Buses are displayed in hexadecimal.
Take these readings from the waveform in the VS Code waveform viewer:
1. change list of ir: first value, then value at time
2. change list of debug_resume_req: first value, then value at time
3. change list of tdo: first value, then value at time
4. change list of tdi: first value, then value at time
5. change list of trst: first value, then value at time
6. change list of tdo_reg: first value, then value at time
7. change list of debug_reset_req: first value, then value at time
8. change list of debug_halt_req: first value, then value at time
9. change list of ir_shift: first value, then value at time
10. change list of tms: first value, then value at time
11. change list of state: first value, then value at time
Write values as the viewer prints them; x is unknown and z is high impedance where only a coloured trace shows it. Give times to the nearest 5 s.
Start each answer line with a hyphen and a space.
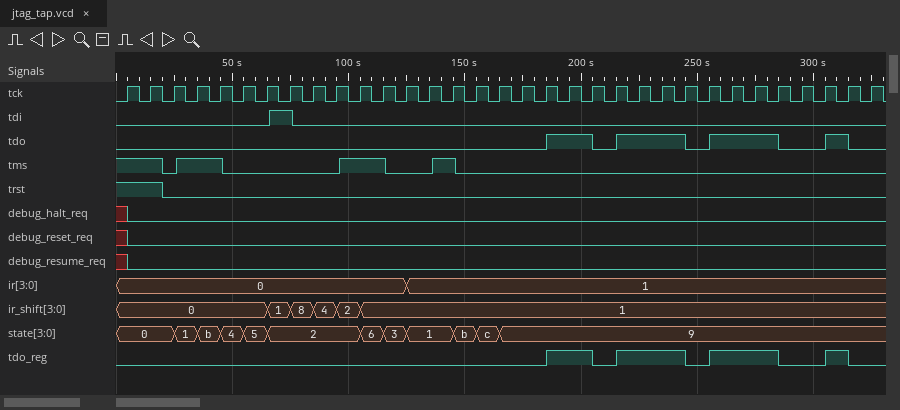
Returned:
- 0, 1 at 125 s
- x, 0 at 5 s
- 0, 1 at 185 s, 0 at 205 s, 1 at 215 s, 0 at 245 s, 1 at 255 s, 0 at 285 s, 1 at 305 s, 0 at 315 s
- 0, 1 at 65 s, 0 at 75 s
- 1, 0 at 20 s
- 0, 1 at 185 s, 0 at 205 s, 1 at 215 s, 0 at 245 s, 1 at 255 s, 0 at 285 s, 1 at 305 s, 0 at 315 s
- x, 0 at 5 s
- x, 0 at 5 s
- 0, 1 at 65 s, 8 at 75 s, 4 at 85 s, 2 at 95 s, 1 at 105 s
- 1, 0 at 20 s, 1 at 25 s, 0 at 45 s, 1 at 95 s, 0 at 115 s, 1 at 135 s, 0 at 145 s
- 0, 1 at 25 s, b at 35 s, 4 at 45 s, 5 at 55 s, 2 at 65 s, 6 at 105 s, 3 at 115 s, 1 at 125 s, b at 145 s, c at 155 s, 9 at 165 s
